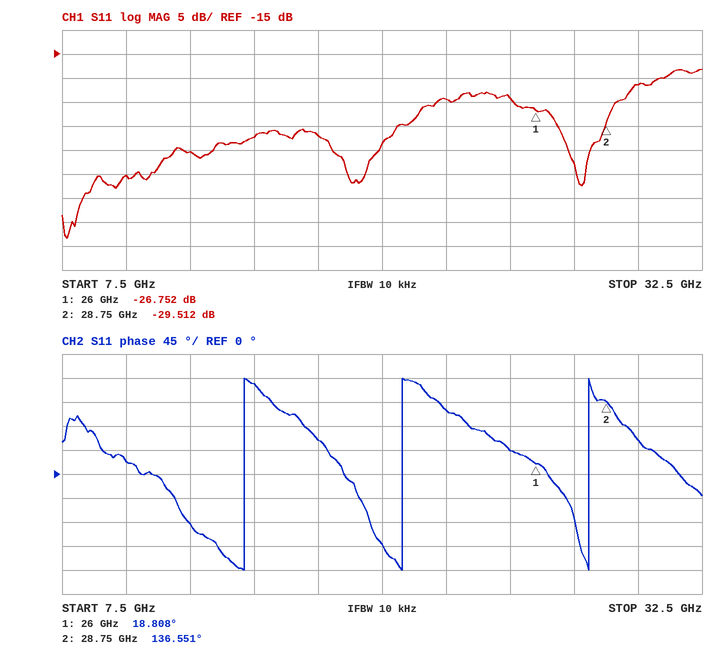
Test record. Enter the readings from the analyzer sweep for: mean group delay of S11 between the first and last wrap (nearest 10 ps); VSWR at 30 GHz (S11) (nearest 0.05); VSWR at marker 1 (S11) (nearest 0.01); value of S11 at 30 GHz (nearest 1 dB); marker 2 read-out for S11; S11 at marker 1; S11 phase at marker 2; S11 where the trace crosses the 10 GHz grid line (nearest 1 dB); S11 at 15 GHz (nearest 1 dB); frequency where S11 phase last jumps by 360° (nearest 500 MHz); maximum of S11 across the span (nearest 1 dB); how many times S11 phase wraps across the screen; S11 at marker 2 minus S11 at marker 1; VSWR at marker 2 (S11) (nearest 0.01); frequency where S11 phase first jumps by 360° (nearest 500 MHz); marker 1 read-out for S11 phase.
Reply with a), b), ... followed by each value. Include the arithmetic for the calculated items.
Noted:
a) 2 cycles / (28.0 GHz − 14.5 GHz) ≈ 148 ps, so 150 ps to the nearest 10 ps
b) |Γ| = 10^(-21/20) = 0.0891; VSWR = (1 + 0.0891)/(1 − 0.0891) ≈ 1.20
c) (1 + 0.0460)/(1 − 0.0460) ≈ 1.10
d) -21 dB
e) -29.512 dB
f) -26.752 dB
g) 136.551°
h) -40 dB
i) -32 dB
j) 28.0 GHz
k) -18 dB
l) 3
m) -29.512 − (-26.752) = -2.760 dB
n) (1 + 0.0335)/(1 − 0.0335) ≈ 1.07
o) 14.5 GHz
p) 18.808°
